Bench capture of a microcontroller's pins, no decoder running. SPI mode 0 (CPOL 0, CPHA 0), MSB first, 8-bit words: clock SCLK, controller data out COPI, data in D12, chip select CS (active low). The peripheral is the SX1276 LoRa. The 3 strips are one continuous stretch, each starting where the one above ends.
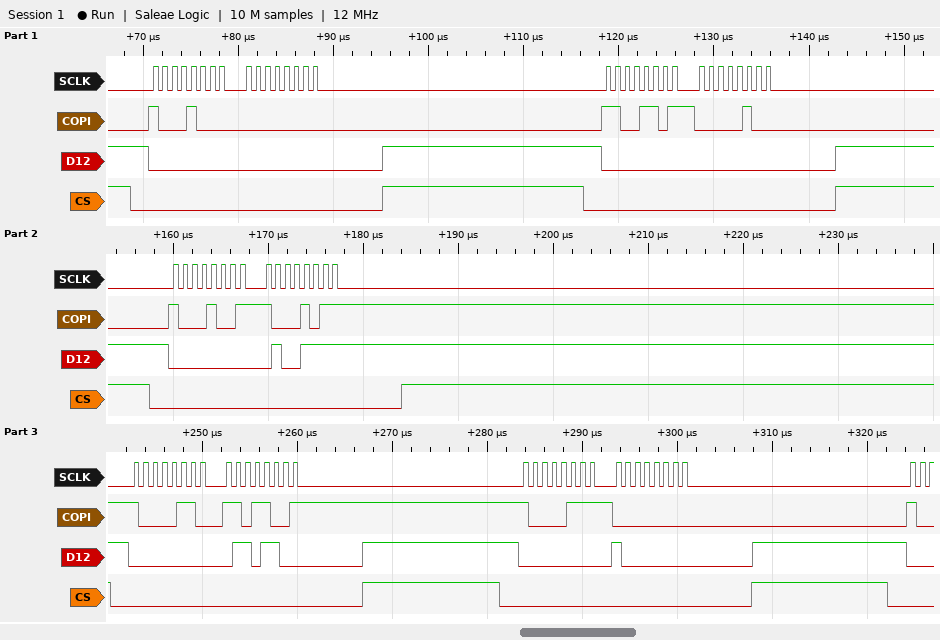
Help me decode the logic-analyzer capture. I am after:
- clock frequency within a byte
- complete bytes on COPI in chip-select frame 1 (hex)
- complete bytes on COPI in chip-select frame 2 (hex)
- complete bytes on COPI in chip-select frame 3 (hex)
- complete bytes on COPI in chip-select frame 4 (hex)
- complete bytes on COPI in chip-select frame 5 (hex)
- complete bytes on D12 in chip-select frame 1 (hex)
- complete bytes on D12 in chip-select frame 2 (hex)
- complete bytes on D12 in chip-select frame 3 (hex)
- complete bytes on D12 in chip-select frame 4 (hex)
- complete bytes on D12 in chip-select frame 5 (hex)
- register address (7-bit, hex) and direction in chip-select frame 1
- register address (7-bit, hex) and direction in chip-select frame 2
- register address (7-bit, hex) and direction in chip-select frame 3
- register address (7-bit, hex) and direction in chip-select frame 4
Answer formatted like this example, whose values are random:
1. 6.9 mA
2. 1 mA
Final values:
1. 1 MHz
2. 88 00
3. CD 04
4. 89 8B
5. 86 D9
6. 87 00
7. 00 00
8. 00 00
9. 00 4F
10. 00 6C
11. 00 80
12. 0x08 write
13. 0x4D write
14. 0x09 write
15. 0x06 write
